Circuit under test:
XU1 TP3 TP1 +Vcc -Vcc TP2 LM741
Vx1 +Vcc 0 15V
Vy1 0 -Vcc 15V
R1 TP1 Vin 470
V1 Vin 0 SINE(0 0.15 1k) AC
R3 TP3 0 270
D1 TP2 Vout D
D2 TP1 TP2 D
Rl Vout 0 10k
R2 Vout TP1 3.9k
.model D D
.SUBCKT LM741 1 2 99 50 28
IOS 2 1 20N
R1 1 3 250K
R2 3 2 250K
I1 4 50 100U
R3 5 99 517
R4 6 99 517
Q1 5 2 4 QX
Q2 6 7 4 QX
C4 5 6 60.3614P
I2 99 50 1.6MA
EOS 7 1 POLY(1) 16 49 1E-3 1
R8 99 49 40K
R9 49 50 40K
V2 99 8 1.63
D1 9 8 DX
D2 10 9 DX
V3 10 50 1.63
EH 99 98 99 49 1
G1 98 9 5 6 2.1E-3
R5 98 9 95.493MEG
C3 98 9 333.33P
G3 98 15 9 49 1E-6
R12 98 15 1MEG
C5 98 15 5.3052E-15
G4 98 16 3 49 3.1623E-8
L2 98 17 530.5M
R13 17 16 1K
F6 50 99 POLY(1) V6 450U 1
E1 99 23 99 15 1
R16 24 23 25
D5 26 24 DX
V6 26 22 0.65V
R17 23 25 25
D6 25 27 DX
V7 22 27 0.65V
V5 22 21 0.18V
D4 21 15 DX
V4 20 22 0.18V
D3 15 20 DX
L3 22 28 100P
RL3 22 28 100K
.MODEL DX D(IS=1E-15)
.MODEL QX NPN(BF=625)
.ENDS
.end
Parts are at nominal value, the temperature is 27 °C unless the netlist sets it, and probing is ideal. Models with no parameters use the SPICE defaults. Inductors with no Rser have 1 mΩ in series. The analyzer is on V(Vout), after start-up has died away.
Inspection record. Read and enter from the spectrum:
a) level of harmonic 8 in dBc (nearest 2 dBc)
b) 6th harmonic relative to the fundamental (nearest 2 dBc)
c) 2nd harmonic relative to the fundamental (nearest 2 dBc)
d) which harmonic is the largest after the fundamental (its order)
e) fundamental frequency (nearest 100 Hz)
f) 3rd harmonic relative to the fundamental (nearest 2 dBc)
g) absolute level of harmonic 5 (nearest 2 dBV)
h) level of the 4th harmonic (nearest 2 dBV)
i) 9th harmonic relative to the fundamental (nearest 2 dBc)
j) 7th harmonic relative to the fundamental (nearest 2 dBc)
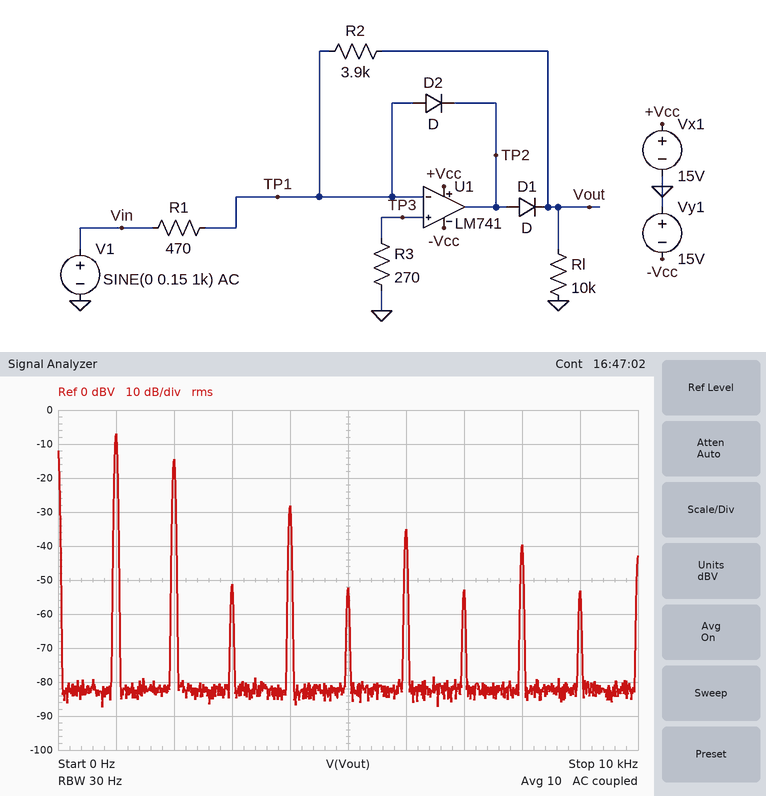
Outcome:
-32 dBc
-28 dBc
-8 dBc
2
1.0 kHz
-44 dBc
-52 dBV
-28 dBV
-46 dBc
-46 dBc
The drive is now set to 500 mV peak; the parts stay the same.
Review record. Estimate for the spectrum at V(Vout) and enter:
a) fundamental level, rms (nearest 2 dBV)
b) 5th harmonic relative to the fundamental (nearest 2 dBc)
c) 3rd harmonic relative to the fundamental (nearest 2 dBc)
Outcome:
4 dBV
-54 dBc
-54 dBc
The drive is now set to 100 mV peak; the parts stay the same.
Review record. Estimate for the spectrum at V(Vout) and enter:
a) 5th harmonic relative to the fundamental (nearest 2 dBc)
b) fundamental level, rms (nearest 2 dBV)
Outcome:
-42 dBc
-10 dBV
